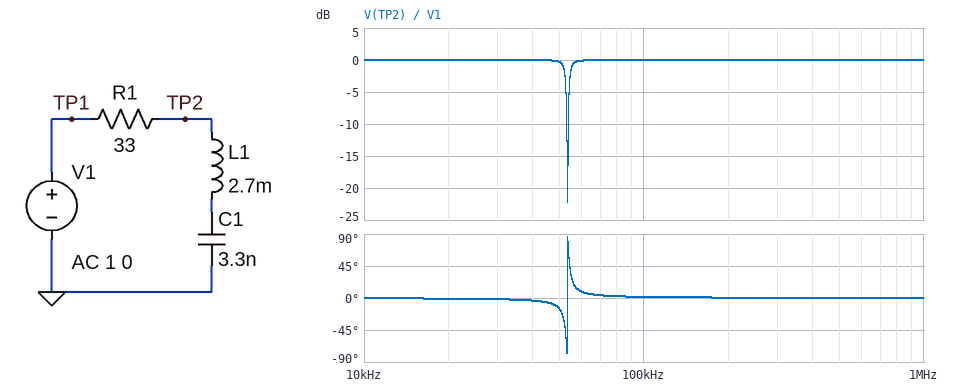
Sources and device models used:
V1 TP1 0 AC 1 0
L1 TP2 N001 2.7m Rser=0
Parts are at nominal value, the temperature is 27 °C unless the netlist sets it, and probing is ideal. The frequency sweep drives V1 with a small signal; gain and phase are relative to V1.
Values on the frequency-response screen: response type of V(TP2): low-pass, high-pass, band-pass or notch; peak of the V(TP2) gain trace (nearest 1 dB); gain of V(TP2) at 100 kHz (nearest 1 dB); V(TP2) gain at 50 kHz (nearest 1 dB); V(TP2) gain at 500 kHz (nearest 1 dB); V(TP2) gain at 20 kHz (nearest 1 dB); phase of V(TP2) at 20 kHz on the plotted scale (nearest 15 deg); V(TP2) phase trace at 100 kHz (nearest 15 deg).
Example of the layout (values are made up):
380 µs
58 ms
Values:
notch
0 dB
0 dB
0 dB
0 dB
0 dB
0 deg
0 deg
